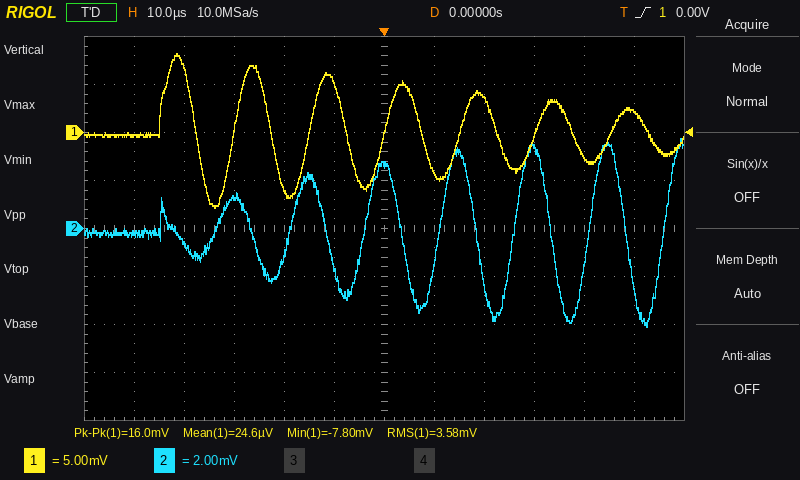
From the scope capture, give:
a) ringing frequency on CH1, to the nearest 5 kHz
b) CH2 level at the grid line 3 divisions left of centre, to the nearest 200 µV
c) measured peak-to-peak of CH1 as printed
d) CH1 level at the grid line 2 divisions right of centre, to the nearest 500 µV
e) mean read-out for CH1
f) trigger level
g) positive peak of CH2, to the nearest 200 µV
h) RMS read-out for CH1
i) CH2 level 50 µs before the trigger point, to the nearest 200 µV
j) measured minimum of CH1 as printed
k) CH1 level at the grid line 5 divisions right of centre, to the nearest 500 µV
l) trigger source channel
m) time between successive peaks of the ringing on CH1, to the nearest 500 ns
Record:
65 kHz
1.4 mV
16.0 mV
3.5 mV
24.6 µV
0.00 V
3.8 mV
3.58 mV
-200 µV
-7.80 mV
2.0 mV
CH1
15.0 µs
